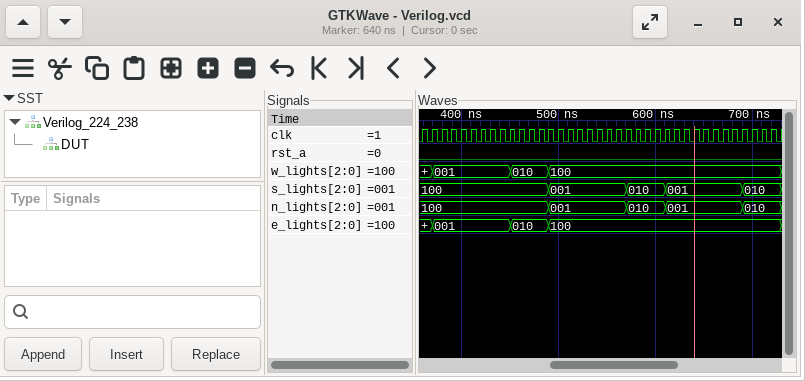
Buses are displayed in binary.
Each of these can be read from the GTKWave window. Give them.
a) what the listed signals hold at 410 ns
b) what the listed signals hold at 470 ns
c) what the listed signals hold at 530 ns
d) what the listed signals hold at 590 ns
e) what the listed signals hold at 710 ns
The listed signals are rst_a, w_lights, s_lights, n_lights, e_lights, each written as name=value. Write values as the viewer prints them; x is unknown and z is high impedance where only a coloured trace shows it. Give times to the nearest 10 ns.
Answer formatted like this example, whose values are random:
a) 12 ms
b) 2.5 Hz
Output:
a) rst_a=0, w_lights=001, s_lights=100, n_lights=100, e_lights=001
b) rst_a=0, w_lights=010, s_lights=100, n_lights=100, e_lights=010
c) rst_a=0, w_lights=100, s_lights=001, n_lights=001, e_lights=100
d) rst_a=0, w_lights=100, s_lights=010, n_lights=010, e_lights=100
e) rst_a=0, w_lights=100, s_lights=010, n_lights=010, e_lights=100
